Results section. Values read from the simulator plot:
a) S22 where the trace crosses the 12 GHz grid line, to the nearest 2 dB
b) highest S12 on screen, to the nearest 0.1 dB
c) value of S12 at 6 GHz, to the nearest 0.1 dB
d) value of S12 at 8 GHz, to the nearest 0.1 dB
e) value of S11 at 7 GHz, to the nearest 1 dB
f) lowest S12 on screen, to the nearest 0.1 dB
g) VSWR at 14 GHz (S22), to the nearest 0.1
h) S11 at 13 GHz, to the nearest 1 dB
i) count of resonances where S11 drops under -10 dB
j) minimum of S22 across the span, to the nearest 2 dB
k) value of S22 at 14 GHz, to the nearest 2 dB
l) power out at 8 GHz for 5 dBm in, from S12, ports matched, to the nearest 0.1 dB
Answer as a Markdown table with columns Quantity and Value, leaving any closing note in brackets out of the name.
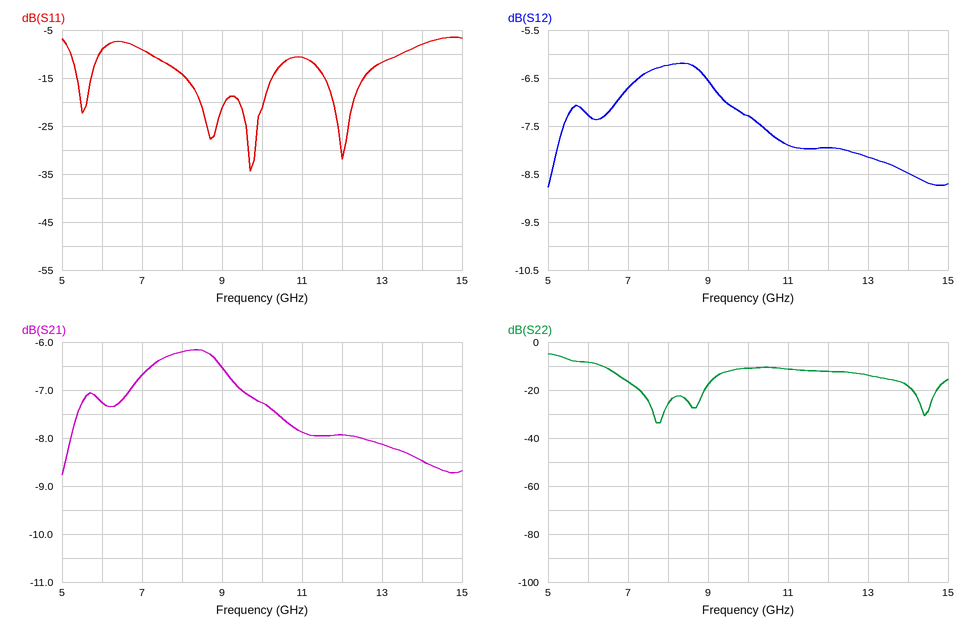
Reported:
| Quantity | Value |
|---|---|
| S22 where the trace crosses the 12 GHz grid line, to the nearest 2 dB | -12 dB |
| highest S12 on screen, to the nearest 0.1 dB | -6.2 dB |
| value of S12 at 6 GHz, to the nearest 0.1 dB | -7.3 dB |
| value of S12 at 8 GHz, to the nearest 0.1 dB | -6.2 dB |
| value of S11 at 7 GHz, to the nearest 1 dB | -9 dB |
| lowest S12 on screen, to the nearest 0.1 dB | -8.8 dB |
| VSWR at 14 GHz (S22), to the nearest 0.1 | 1.3 |
| S11 at 13 GHz, to the nearest 1 dB | -12 dB |
| count of resonances where S11 drops under -10 dB | 4 |
| minimum of S22 across the span, to the nearest 2 dB | -34 dB |
| value of S22 at 14 GHz, to the nearest 2 dB | -18 dB |
| power out at 8 GHz for 5 dBm in, from S12, ports matched, to the nearest 0.1 dB | -1.2 dBm |
